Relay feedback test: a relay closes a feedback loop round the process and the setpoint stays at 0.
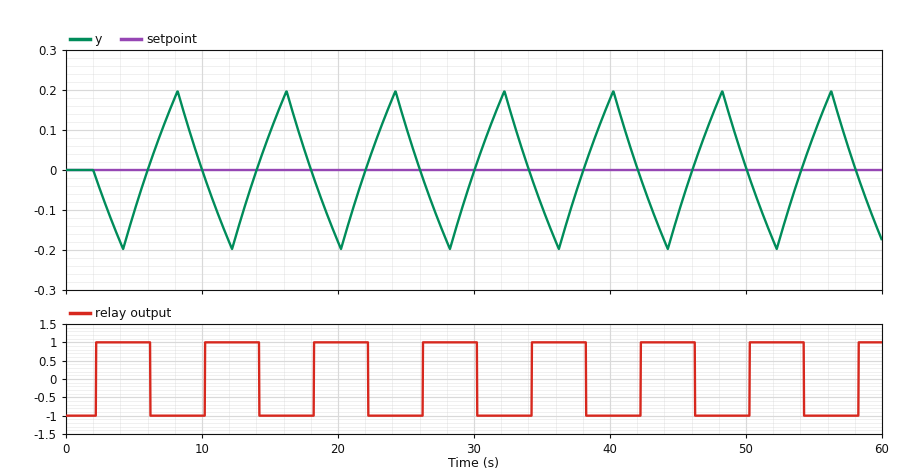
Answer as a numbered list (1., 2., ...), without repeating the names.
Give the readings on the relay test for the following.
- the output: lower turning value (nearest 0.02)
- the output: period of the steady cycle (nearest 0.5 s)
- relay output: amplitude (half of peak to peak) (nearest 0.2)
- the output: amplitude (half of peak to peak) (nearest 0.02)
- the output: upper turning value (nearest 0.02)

1. -0.20
2. 8.0 s
3. 1.0
4. 0.20
5. 0.20
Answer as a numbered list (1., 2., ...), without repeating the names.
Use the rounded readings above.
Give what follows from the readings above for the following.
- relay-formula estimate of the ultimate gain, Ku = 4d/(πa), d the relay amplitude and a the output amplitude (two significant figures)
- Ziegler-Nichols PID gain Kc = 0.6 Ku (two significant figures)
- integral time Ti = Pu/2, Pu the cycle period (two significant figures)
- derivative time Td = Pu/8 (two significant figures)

1. 6.4
2. 3.8
3. 4.0 s
4. 1.0 s
